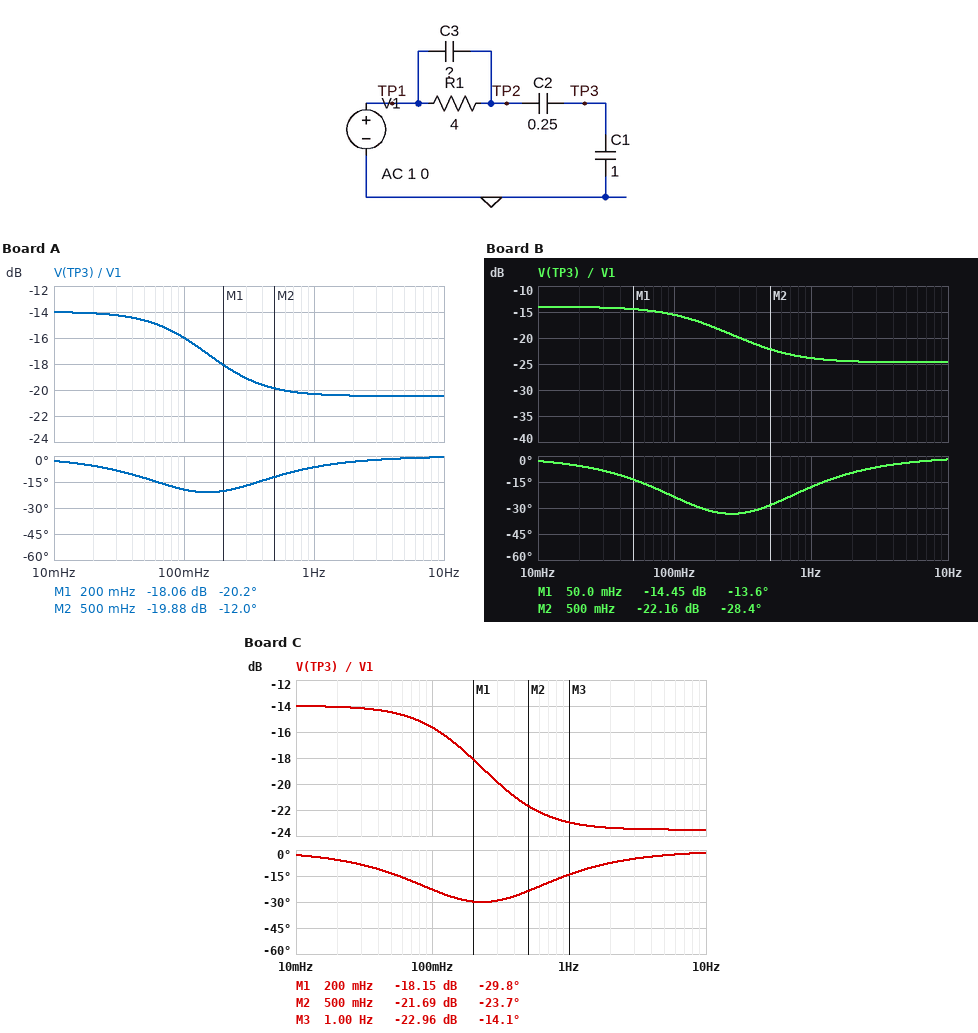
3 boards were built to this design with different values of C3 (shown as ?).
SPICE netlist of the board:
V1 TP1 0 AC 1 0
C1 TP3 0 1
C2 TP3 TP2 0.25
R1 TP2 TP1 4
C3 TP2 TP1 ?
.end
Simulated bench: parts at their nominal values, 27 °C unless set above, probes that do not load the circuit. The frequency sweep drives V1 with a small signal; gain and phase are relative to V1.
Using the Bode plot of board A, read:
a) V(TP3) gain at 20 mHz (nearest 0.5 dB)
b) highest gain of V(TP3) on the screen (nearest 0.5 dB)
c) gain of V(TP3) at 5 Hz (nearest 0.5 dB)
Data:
-14.0 dB
-14.0 dB
-20.5 dB
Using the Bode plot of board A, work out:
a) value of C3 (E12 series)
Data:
180 mF
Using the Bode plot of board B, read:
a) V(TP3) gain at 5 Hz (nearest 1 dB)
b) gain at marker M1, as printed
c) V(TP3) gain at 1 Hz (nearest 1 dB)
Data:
-25 dB
-14.45 dB
-24 dB
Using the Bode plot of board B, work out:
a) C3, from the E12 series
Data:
82 mF
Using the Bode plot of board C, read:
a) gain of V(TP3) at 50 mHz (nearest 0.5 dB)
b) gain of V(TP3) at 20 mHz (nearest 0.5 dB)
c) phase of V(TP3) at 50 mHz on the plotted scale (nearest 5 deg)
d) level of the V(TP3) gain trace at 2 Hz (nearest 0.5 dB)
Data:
-14.5 dB
-14.0 dB
-15 deg
-23.5 dB
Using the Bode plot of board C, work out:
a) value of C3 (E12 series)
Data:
100 mF
